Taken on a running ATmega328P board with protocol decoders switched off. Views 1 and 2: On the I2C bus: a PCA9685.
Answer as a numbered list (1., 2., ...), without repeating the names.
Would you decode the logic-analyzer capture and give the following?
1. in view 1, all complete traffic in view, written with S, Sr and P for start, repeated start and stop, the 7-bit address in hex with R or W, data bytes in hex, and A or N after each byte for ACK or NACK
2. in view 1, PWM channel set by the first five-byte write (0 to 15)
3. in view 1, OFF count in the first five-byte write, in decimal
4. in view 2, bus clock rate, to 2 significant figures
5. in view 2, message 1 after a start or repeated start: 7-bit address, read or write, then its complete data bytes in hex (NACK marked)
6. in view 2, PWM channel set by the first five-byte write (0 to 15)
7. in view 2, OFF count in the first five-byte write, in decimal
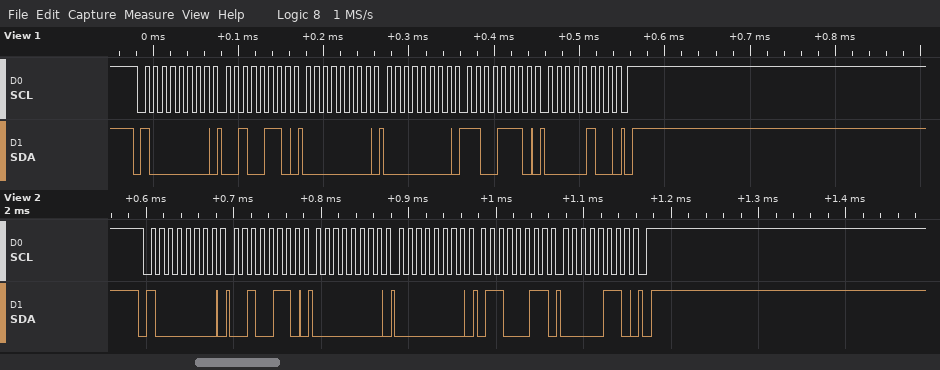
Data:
1. S 40W A 26 A 00 A 00 A CE A 04 A P
2. 8
3. 1230
4. 100 kHz
5. 0x40 write: 26 00 00 63 06
6. 8
7. 1635
